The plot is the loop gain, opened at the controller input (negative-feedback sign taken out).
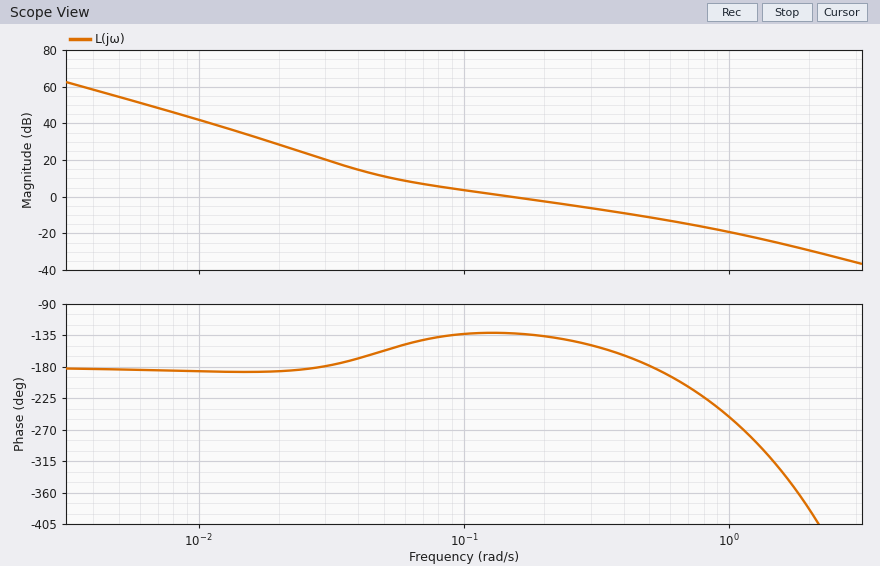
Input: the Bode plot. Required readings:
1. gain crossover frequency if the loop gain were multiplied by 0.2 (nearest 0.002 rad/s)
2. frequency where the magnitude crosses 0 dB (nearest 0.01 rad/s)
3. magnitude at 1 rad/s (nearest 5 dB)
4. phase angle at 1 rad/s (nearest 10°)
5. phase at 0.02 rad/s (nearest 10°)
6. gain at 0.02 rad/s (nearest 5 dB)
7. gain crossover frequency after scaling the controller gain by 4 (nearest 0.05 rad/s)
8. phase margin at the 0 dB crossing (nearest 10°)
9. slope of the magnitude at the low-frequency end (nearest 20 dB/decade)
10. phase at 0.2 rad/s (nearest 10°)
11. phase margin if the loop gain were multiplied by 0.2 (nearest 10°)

0.042 rad/s
0.15 rad/s
-20 dB
-250°
-190°
30 dB
0.55 rad/s
50°
-40 dB/decade
-140°
10°
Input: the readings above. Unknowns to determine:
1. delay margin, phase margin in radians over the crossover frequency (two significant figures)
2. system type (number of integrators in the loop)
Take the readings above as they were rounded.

5.8 s
2
